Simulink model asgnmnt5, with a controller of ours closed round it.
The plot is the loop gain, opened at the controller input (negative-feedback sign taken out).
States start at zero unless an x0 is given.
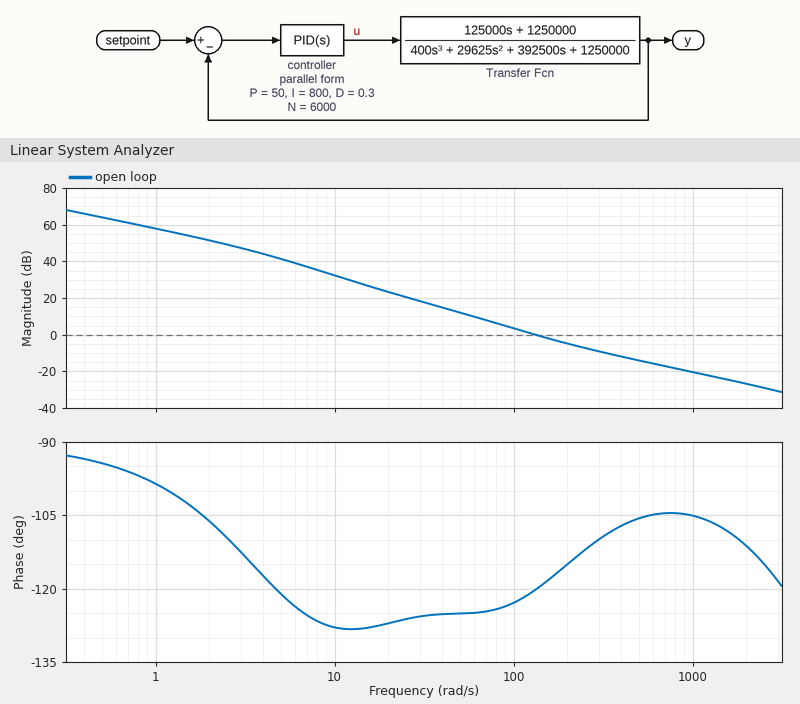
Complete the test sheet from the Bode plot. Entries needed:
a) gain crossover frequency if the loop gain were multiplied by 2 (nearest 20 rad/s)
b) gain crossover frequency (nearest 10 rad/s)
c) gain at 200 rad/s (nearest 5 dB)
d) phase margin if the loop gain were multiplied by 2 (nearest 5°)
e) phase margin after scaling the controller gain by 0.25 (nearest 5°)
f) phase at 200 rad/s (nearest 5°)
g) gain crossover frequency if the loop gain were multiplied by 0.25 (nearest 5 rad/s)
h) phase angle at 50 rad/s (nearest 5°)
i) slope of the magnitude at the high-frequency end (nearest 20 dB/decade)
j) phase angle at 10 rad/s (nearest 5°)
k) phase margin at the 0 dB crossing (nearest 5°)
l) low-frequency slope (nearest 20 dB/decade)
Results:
220 rad/s
130 rad/s
-5 dB
65°
55°
-115°
50 rad/s
-125°
-20 dB/decade
-130°
60°
-20 dB/decade
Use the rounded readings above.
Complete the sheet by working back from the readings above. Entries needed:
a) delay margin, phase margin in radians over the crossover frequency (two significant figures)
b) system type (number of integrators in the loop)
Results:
0.0081 s
1
